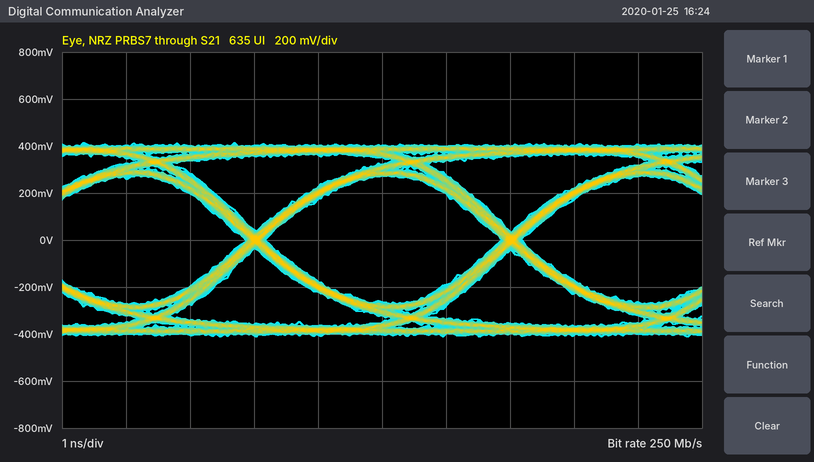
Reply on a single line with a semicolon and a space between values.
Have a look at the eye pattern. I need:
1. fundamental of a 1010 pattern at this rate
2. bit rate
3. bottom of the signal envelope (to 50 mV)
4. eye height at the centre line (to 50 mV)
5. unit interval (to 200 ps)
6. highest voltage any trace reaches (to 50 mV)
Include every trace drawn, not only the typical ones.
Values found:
125 MHz; 250 Mb/s; -400 mV; 550 mV; 4.0 ns; 400 mV
